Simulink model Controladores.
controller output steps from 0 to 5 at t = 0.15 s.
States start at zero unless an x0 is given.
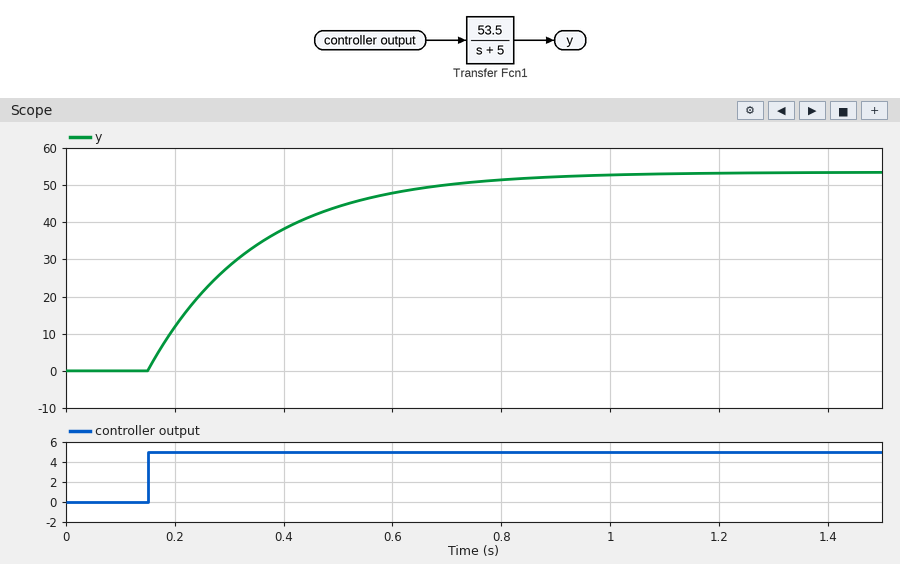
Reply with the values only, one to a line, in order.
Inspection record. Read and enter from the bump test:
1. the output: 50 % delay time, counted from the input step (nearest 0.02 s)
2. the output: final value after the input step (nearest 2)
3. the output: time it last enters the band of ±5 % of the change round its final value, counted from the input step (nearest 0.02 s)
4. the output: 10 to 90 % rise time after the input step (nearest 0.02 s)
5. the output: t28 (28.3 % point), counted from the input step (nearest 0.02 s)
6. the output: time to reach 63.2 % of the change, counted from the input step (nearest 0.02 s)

0.14 s
54
0.60 s
0.44 s
0.06 s
0.20 s
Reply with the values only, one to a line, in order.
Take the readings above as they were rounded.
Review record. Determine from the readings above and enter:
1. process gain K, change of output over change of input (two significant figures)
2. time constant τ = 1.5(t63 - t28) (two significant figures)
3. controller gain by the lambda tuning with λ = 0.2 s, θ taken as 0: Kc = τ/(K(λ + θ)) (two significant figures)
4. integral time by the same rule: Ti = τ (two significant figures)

11
0.21 s
0.095
0.21 s
